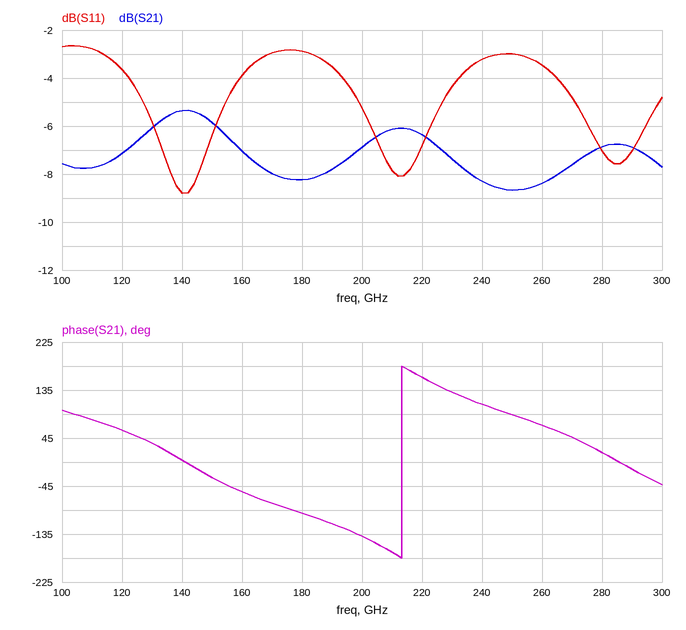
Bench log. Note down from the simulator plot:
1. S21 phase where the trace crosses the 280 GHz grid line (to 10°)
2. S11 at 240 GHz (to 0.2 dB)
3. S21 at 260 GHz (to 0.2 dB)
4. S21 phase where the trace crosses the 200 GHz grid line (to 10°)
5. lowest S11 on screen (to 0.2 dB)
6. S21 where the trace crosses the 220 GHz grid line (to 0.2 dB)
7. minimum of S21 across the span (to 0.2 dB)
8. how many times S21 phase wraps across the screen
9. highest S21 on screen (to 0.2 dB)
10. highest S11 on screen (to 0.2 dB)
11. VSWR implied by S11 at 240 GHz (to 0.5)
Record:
20°
-3.2 dB
-8.4 dB
-140°
-8.8 dB
-6.4 dB
-8.6 dB
1
-5.4 dB
-2.6 dB
5.5
